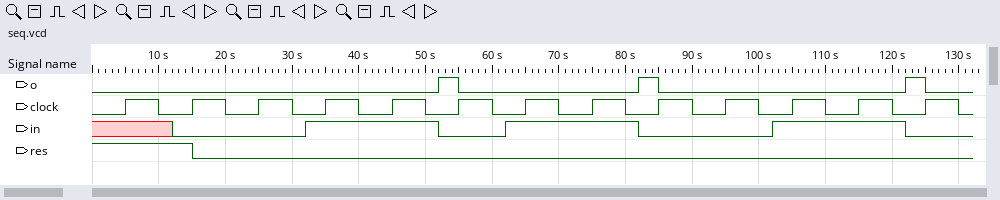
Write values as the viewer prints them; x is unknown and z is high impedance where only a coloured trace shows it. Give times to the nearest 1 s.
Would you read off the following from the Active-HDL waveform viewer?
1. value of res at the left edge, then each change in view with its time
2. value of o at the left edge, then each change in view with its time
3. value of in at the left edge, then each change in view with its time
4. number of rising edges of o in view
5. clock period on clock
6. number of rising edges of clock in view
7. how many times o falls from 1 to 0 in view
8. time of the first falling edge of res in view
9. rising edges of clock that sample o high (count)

1, 0 at 15 s
0, 1 at 52 s, 0 at 55 s, 1 at 82 s, 0 at 85 s, 1 at 122 s, 0 at 125 s
x, 0 at 12 s, 1 at 32 s, 0 at 52 s, 1 at 62 s, 0 at 82 s, 1 at 102 s, 0 at 122 s
3
10 s
13
3
15 s
3
